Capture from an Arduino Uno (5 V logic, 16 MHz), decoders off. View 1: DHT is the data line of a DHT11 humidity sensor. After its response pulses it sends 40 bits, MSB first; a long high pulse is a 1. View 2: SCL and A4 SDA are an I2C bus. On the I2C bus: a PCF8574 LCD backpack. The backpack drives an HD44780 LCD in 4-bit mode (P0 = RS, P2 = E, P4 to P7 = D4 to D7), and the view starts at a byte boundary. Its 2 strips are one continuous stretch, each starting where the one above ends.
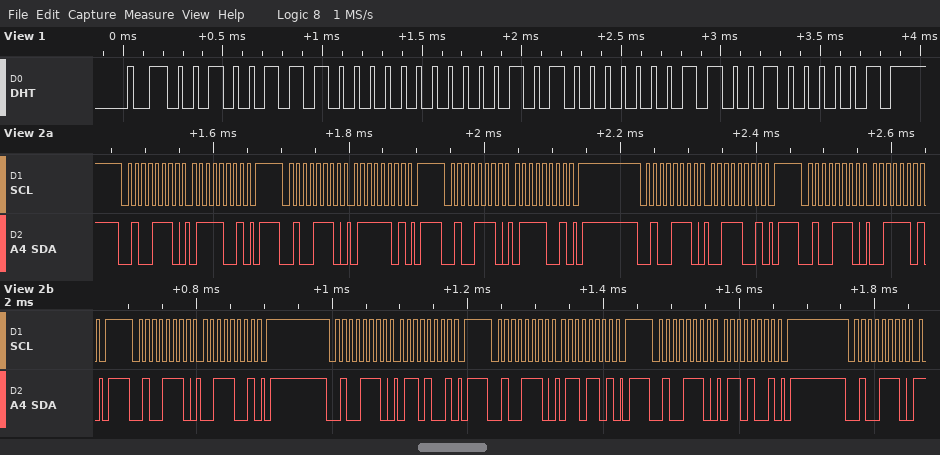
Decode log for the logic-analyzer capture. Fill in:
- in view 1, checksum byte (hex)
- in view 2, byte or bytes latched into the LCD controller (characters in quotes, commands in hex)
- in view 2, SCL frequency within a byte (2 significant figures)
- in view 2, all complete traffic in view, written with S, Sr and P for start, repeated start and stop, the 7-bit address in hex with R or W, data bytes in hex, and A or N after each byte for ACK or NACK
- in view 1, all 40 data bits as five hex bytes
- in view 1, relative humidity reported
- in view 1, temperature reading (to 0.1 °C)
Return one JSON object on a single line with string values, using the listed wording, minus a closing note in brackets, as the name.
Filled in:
{"in view 1, checksum byte": "0x41", "in view 2, byte or bytes latched into the LCD controller": "'s'", "in view 2, SCL frequency within a byte": "100 kHz", "in view 2, all complete traffic in view, written with S, Sr and P for start, repeated start and stop, the 7-bit address in hex with R or W, data bytes in hex, and A or N after each byte for ACK or NACK": "S 27W A 79 A P S 27W A 7D A P S 27W A 79 A P S 27W A 39 A P S 27W A 3D A P S 27W A 39 A P S 27W A 69 A P S 27W A 6D A P S 27W A 69 A P S 27W A", "in view 1, all 40 data bits as five hex bytes": "27 00 14 06 41", "in view 1, relative humidity reported": "39 %", "in view 1, temperature reading": "20.6 °C"}
